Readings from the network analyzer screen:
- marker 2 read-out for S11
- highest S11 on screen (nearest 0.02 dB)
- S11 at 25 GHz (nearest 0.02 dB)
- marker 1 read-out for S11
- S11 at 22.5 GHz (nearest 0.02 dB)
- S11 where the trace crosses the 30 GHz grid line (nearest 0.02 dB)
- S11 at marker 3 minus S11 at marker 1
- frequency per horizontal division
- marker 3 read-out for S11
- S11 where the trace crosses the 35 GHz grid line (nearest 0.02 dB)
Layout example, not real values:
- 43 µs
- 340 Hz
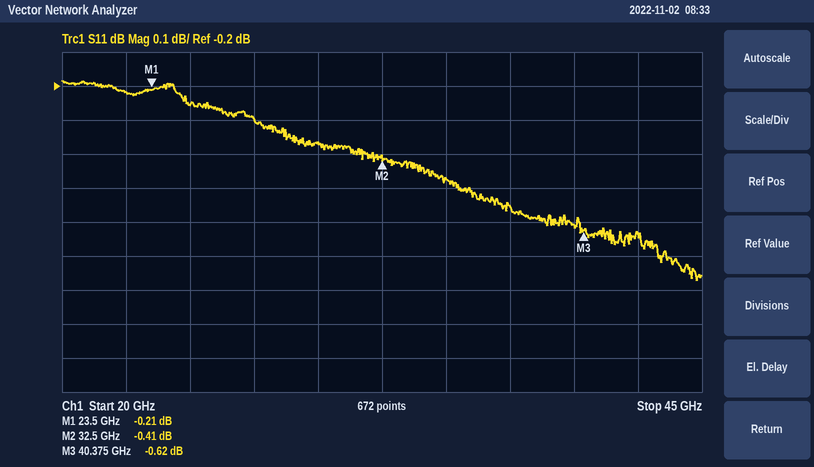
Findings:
- -0.41 dB
- -0.18 dB
- -0.26 dB
- -0.21 dB
- -0.22 dB
- -0.36 dB
- -0.41 dB
- 2.5 GHz
- -0.62 dB
- -0.48 dB
